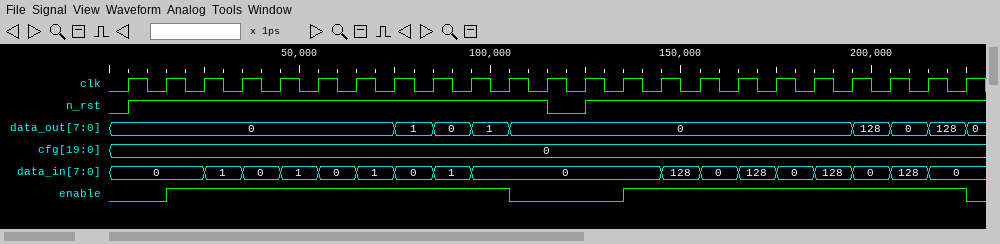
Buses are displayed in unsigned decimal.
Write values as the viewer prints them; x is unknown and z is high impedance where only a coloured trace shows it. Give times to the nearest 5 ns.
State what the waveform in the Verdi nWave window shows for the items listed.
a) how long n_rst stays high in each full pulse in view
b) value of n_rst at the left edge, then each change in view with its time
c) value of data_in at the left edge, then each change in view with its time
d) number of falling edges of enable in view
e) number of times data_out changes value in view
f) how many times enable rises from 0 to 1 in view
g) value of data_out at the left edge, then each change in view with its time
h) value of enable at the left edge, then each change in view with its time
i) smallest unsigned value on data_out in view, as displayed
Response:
110 ns
0, 1 at 5 ns, 0 at 115 ns, 1 at 125 ns
0, 1 at 25 ns, 0 at 35 ns, 1 at 45 ns, 0 at 55 ns, 1 at 65 ns, 0 at 75 ns, 1 at 85 ns, 0 at 95 ns, 128 at 145 ns, 0 at 155 ns, 128 at 165 ns, 0 at 175 ns, 128 at 185 ns, 0 at 195 ns, 128 at 205 ns, 0 at 215 ns
2
8
2
0, 1 at 75 ns, 0 at 85 ns, 1 at 95 ns, 0 at 105 ns, 128 at 195 ns, 0 at 205 ns, 128 at 215 ns, 0 at 225 ns
0, 1 at 15 ns, 0 at 105 ns, 1 at 135 ns, 0 at 225 ns
0
